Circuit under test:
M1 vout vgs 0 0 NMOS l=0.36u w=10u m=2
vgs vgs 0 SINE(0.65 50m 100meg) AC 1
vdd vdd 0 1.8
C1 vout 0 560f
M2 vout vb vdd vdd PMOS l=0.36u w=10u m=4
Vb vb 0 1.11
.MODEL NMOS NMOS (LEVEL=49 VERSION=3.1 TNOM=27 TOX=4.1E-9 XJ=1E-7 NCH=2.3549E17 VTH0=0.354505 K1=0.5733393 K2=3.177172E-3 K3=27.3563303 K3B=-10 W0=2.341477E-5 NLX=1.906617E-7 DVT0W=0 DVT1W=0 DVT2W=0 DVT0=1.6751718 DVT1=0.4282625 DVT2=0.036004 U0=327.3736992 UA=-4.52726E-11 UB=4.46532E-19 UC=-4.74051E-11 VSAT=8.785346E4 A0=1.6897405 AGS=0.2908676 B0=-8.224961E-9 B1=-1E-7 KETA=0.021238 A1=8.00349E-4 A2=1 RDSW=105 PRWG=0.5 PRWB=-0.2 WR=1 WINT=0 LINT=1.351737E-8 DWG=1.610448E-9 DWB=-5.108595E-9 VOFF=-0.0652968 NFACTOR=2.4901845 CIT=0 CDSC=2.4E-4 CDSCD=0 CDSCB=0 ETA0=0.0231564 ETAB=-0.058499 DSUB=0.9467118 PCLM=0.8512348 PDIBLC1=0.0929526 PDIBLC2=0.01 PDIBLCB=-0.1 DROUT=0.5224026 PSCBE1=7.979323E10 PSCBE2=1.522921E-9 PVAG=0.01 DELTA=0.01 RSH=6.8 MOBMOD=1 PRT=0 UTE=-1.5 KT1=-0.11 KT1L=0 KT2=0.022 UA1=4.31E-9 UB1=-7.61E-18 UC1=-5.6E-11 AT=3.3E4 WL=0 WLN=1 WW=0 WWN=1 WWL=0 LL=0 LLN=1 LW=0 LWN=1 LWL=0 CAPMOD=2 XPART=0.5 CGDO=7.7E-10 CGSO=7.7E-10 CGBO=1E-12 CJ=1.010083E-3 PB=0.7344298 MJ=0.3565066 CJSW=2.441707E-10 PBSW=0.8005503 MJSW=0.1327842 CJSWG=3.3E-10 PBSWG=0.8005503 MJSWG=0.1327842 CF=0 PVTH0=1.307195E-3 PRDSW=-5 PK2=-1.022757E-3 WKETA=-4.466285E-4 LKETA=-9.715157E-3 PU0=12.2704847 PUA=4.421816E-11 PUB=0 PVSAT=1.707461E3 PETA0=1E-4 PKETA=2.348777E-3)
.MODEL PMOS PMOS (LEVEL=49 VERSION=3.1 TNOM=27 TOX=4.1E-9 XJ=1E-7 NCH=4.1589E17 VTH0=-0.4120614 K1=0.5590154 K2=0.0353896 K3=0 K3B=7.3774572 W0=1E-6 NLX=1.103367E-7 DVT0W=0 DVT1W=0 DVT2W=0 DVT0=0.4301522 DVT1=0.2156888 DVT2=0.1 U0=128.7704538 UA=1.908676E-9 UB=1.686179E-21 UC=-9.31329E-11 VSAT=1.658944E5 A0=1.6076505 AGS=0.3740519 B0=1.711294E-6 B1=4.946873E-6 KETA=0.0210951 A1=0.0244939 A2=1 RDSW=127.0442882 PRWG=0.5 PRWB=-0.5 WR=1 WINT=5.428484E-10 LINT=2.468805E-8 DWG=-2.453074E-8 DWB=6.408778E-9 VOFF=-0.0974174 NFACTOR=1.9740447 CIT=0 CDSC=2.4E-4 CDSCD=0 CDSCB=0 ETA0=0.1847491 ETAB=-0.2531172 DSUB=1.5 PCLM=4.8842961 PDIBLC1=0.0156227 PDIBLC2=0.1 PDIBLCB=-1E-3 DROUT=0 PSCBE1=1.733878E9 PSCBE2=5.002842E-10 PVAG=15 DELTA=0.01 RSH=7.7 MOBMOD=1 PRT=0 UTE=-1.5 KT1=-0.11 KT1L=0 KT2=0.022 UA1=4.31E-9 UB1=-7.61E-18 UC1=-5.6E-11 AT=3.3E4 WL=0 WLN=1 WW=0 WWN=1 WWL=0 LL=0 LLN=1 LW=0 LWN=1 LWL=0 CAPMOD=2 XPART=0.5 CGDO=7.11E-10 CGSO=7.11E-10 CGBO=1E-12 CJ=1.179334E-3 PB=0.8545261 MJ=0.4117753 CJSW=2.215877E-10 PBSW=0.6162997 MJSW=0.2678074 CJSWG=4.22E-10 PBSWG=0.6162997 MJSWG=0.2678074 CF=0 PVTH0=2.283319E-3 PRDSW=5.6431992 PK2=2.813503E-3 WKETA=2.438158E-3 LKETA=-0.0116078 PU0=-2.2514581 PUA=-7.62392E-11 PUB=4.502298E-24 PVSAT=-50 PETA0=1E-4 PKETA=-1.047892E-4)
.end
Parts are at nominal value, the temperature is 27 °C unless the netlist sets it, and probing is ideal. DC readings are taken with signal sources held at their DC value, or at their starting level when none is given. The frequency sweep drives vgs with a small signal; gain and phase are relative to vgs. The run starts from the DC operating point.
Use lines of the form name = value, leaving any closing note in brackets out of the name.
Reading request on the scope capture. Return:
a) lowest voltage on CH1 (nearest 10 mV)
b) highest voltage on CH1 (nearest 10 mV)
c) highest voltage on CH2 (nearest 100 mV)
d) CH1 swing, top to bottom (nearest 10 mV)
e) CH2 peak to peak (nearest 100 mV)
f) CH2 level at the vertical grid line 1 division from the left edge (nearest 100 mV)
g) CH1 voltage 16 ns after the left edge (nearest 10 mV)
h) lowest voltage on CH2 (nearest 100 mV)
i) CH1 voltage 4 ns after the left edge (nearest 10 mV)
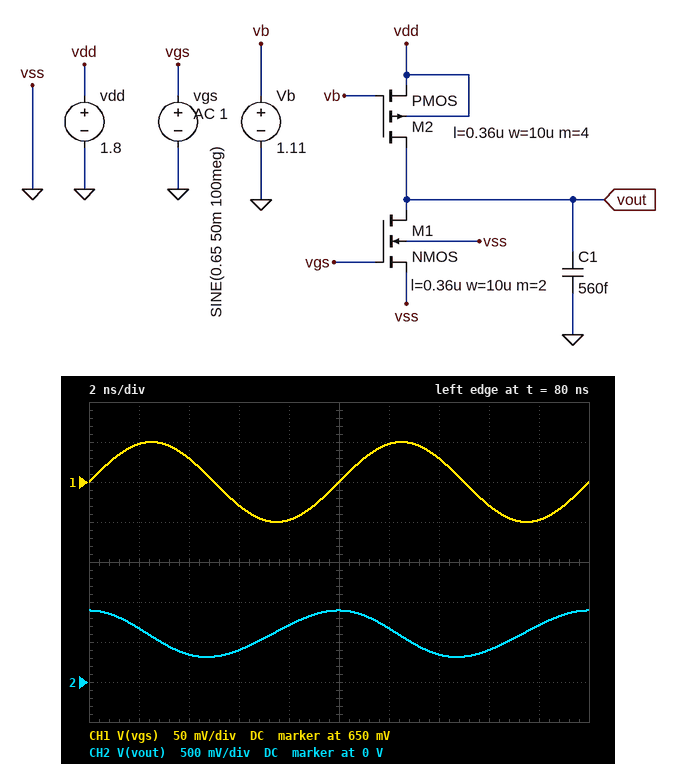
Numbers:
lowest voltage on CH1 = 600 mV
highest voltage on CH1 = 700 mV
highest voltage on CH2 = 900 mV
CH1 swing, top to bottom = 100 mV
CH2 peak to peak = 600 mV
CH2 level at the vertical grid line 1 division from the left edge = 700 mV
CH1 voltage 16 ns after the left edge = 620 mV
lowest voltage on CH2 = 300 mV
CH1 voltage 4 ns after the left edge = 680 mV
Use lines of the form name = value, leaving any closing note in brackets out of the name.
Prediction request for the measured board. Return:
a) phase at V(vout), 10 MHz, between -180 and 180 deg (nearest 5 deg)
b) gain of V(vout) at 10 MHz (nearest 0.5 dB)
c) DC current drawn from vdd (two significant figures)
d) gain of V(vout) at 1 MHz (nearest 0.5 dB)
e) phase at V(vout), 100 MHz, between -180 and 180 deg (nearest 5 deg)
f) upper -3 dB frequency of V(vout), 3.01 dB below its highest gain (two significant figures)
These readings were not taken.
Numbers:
phase at V(vout), 10 MHz, between -180 and 180 deg = 135 deg
gain of V(vout) at 10 MHz = 32.5 dB
DC current drawn from vdd = 190 µA
gain of V(vout) at 1 MHz = 35.5 dB
phase at V(vout), 100 MHz, between -180 and 180 deg = 95 deg
upper -3 dB frequency of V(vout), 3.01 dB below its highest gain = 9.8 MHz
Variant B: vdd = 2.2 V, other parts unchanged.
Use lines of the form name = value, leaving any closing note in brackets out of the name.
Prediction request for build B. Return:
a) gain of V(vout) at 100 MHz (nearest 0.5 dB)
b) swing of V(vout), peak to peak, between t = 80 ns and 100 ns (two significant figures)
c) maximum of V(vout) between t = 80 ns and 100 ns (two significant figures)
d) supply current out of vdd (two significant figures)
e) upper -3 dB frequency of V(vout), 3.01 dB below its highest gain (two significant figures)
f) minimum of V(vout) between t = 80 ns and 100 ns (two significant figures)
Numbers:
gain of V(vout) at 100 MHz = -4.5 dB
swing of V(vout), peak to peak, between t = 80 ns and 100 ns = 60 mV
maximum of V(vout) between t = 80 ns and 100 ns = 2.2 V
supply current out of vdd = 220 µA
upper -3 dB frequency of V(vout), 3.01 dB below its highest gain = 1.0 GHz
minimum of V(vout) between t = 80 ns and 100 ns = 2.1 V
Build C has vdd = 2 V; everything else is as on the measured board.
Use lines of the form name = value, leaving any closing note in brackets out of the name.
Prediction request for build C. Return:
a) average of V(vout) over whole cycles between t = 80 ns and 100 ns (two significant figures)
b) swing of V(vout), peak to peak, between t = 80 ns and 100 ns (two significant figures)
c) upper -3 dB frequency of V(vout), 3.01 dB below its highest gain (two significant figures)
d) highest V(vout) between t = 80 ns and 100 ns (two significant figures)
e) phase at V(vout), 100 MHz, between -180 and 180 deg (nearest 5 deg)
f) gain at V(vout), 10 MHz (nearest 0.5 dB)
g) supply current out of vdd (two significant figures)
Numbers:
average of V(vout) over whole cycles between t = 80 ns and 100 ns = 1.9 V
swing of V(vout), peak to peak, between t = 80 ns and 100 ns = 97 mV
upper -3 dB frequency of V(vout), 3.01 dB below its highest gain = 640 MHz
highest V(vout) between t = 80 ns and 100 ns = 2.0 V
phase at V(vout), 100 MHz, between -180 and 180 deg = 170 deg
gain at V(vout), 10 MHz = -0.5 dB
supply current out of vdd = 220 µA
